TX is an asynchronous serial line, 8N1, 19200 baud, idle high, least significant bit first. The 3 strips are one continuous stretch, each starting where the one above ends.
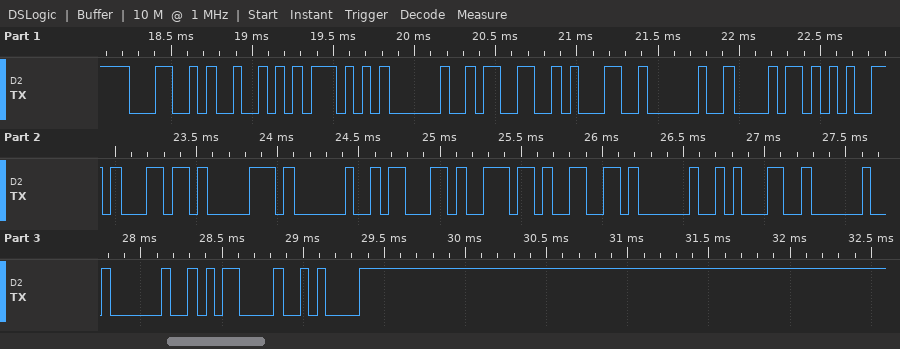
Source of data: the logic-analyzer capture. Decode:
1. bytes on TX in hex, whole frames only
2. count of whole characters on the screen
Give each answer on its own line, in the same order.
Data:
0x4C 0x52 0x57 0x20 0x33 0x31 0x20 0x68 0x65 0x6C 0x70 0x20 0x63 0x6E 0x66 0x20 0x31 0x20 0x20 0x0D 0x0A
21
